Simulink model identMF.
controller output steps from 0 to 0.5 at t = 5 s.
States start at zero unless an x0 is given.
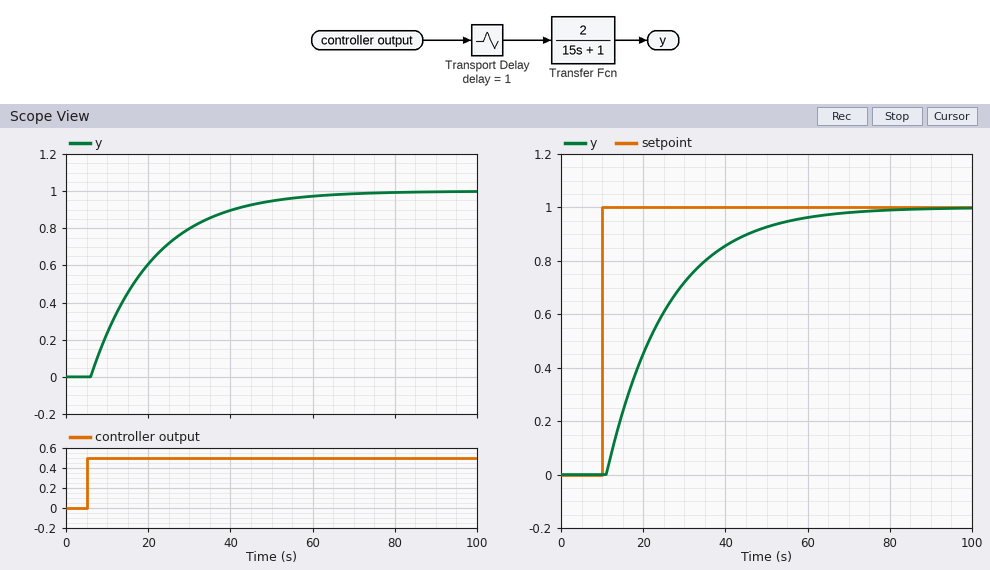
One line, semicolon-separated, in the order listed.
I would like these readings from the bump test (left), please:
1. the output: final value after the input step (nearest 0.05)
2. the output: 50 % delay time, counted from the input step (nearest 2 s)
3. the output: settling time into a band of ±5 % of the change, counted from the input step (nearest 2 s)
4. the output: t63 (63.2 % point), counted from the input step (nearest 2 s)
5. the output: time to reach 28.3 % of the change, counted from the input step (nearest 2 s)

1.00; 12 s; 46 s; 16 s; 6 s
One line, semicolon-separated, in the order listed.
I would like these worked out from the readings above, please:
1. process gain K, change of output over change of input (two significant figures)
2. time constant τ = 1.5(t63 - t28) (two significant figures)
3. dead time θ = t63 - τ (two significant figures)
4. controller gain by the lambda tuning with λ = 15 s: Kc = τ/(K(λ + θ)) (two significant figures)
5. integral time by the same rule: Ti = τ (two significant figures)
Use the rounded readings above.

2.0; 15 s; 1.0 s; 0.47; 15 s
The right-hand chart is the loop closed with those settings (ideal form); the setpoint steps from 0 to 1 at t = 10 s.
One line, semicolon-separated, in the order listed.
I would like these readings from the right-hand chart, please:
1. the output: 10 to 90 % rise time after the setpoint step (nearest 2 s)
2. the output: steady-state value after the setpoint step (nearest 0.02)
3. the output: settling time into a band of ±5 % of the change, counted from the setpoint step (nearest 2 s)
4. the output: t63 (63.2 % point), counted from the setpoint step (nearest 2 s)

32 s; 1.00; 46 s; 16 s
